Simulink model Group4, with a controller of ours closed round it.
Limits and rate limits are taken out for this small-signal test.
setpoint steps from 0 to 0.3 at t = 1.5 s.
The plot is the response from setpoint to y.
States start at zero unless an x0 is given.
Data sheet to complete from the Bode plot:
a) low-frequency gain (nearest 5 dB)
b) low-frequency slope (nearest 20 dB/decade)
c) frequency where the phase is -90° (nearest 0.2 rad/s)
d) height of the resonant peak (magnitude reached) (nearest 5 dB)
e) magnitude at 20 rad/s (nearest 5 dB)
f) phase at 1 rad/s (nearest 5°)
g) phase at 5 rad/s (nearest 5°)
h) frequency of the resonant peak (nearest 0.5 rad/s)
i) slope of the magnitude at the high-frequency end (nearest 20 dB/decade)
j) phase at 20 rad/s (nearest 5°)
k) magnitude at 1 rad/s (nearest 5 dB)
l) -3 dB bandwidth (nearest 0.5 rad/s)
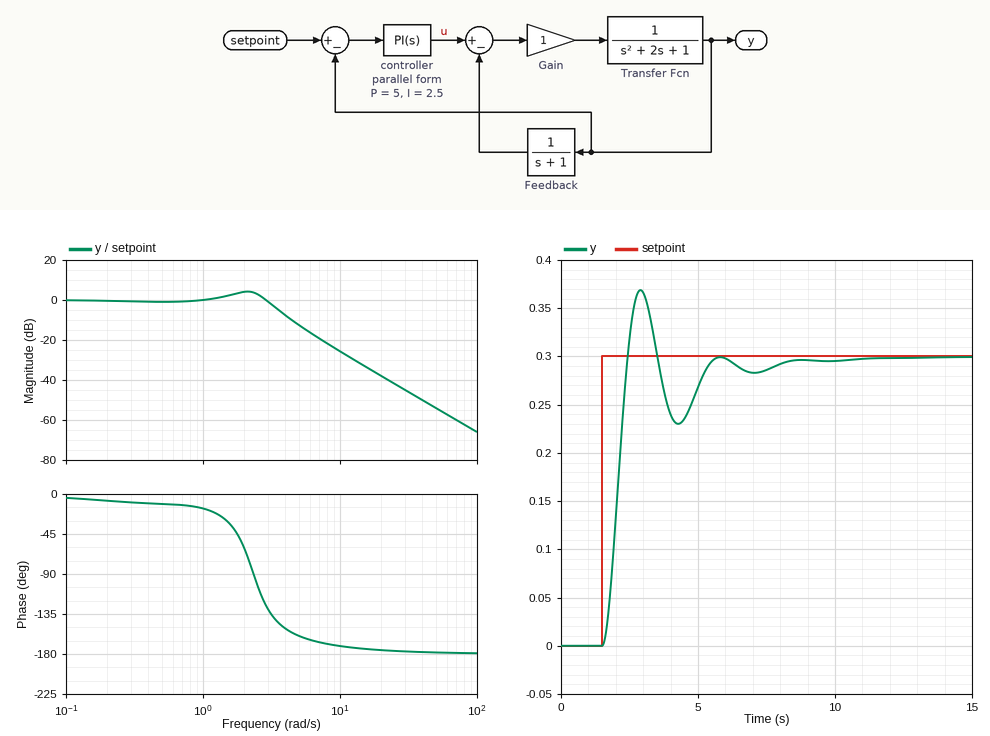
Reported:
0 dB
0 dB/decade
2.4 rad/s
5 dB
-40 dB
-15°
-160°
2.0 rad/s
-40 dB/decade
-175°
0 dB
3.5 rad/s
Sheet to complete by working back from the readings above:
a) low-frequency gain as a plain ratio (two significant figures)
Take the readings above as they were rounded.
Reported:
1.0
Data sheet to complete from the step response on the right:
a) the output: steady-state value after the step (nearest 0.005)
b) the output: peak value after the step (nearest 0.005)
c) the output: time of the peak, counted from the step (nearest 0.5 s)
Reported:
0.300
0.370
1.5 s
